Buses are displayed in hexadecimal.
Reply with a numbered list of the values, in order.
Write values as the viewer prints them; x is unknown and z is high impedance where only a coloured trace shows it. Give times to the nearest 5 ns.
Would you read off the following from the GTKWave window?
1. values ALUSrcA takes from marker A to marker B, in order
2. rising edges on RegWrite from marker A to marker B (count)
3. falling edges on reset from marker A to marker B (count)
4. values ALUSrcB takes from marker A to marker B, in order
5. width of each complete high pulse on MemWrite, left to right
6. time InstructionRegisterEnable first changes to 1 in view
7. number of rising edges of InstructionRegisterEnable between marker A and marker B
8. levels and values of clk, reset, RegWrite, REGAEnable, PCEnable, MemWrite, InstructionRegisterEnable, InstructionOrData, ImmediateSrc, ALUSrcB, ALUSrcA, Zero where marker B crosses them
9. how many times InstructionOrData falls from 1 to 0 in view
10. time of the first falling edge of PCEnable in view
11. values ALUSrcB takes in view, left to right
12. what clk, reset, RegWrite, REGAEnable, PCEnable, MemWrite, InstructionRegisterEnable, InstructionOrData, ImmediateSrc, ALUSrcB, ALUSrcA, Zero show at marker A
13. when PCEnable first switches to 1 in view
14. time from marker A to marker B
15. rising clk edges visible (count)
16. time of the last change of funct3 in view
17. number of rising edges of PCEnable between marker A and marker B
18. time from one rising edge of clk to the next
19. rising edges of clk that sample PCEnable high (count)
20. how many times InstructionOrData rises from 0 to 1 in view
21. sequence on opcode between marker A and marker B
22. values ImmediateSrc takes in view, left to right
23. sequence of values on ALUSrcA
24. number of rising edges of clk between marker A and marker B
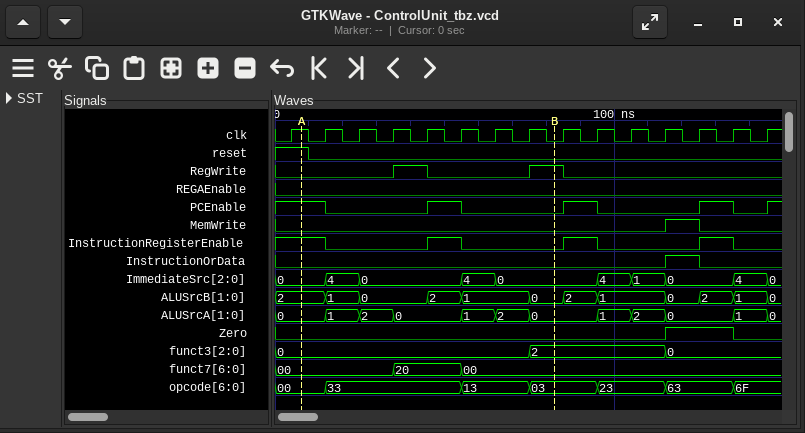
1. 0, 1, 2, 0, 1, 2, 0
2. 2
3. 1
4. 2, 1, 0, 2, 1, 0
5. 10 ns
6. 45 ns
7. 1
8. clk=0, reset=0, RegWrite=1, REGAEnable=0, PCEnable=0, MemWrite=0, InstructionRegisterEnable=0, InstructionOrData=0, ImmediateSrc=0, ALUSrcB=0, ALUSrcA=0, Zero=0
9. 1
10. 15 ns
11. 2, 1, 0, 2, 1, 0, 2, 1, 0, 2, 1, 0
12. clk=1, reset=1, RegWrite=0, REGAEnable=0, PCEnable=1, MemWrite=0, InstructionRegisterEnable=1, InstructionOrData=0, ImmediateSrc=0, ALUSrcB=2, ALUSrcA=0, Zero=0
13. 45 ns
14. 75 ns
15. 15
16. 115 ns
17. 1
18. 10 ns
19. 5
20. 1
21. 00, 33, 13, 03
22. 0, 4, 0, 4, 0, 4, 1, 0, 4, 0
23. 0, 1, 2, 0, 1, 2, 0, 1, 2, 0, 1, 0
24. 7
